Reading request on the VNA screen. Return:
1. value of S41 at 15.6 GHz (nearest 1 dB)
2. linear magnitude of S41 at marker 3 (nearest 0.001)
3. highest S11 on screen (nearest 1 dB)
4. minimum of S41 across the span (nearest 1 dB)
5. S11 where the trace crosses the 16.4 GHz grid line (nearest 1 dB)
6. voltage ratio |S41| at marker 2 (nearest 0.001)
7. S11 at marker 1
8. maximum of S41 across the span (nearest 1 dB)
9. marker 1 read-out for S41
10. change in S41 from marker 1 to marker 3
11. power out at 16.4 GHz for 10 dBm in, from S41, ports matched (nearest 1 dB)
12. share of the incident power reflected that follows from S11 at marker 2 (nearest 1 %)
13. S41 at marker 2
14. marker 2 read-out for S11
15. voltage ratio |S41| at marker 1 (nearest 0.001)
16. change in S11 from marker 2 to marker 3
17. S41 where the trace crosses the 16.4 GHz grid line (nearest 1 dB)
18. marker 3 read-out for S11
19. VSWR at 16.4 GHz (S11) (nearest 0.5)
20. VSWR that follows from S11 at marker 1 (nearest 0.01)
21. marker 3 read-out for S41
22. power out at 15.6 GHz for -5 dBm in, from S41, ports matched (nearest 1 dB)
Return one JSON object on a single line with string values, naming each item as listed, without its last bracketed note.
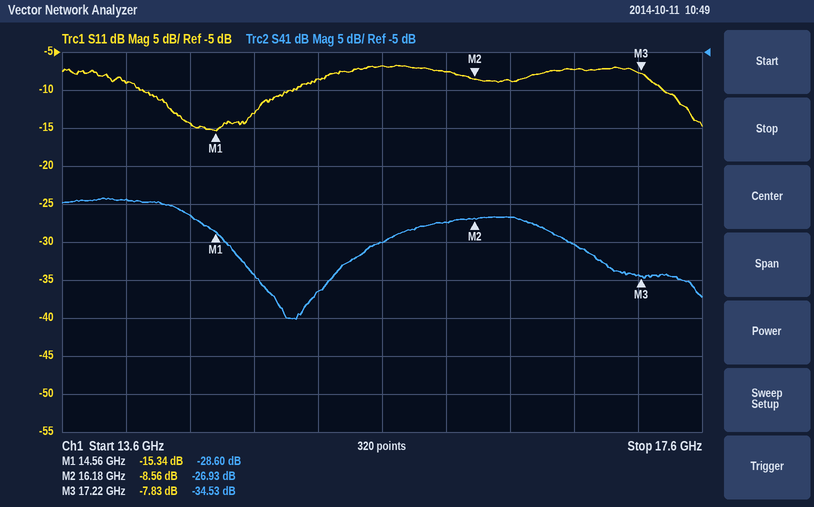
{"value of S41 at 15.6 GHz": "-30 dB", "linear magnitude of S41 at marker 3": "0.019", "highest S11 on screen": "-7 dB", "minimum of S41 across the span": "-40 dB", "S11 where the trace crosses the 16.4 GHz grid line": "-9 dB", "voltage ratio |S41| at marker 2": "0.045", "S11 at marker 1": "-15.34 dB", "maximum of S41 across the span": "-24 dB", "marker 1 read-out for S41": "-28.60 dB", "change in S41 from marker 1 to marker 3": "-5.93 dB", "power out at 16.4 GHz for 10 dBm in, from S41, ports matched": "-17 dBm", "share of the incident power reflected that follows from S11 at marker 2": "14 %", "S41 at marker 2": "-26.93 dB", "marker 2 read-out for S11": "-8.56 dB", "voltage ratio |S41| at marker 1": "0.037", "change in S11 from marker 2 to marker 3": "0.73 dB", "S41 where the trace crosses the 16.4 GHz grid line": "-27 dB", "marker 3 read-out for S11": "-7.83 dB", "VSWR at 16.4 GHz (S11)": "2.0", "VSWR that follows from S11 at marker 1": "1.41", "marker 3 read-out for S41": "-34.53 dB", "power out at 15.6 GHz for -5 dBm in, from S41, ports matched": "-35 dBm"}
